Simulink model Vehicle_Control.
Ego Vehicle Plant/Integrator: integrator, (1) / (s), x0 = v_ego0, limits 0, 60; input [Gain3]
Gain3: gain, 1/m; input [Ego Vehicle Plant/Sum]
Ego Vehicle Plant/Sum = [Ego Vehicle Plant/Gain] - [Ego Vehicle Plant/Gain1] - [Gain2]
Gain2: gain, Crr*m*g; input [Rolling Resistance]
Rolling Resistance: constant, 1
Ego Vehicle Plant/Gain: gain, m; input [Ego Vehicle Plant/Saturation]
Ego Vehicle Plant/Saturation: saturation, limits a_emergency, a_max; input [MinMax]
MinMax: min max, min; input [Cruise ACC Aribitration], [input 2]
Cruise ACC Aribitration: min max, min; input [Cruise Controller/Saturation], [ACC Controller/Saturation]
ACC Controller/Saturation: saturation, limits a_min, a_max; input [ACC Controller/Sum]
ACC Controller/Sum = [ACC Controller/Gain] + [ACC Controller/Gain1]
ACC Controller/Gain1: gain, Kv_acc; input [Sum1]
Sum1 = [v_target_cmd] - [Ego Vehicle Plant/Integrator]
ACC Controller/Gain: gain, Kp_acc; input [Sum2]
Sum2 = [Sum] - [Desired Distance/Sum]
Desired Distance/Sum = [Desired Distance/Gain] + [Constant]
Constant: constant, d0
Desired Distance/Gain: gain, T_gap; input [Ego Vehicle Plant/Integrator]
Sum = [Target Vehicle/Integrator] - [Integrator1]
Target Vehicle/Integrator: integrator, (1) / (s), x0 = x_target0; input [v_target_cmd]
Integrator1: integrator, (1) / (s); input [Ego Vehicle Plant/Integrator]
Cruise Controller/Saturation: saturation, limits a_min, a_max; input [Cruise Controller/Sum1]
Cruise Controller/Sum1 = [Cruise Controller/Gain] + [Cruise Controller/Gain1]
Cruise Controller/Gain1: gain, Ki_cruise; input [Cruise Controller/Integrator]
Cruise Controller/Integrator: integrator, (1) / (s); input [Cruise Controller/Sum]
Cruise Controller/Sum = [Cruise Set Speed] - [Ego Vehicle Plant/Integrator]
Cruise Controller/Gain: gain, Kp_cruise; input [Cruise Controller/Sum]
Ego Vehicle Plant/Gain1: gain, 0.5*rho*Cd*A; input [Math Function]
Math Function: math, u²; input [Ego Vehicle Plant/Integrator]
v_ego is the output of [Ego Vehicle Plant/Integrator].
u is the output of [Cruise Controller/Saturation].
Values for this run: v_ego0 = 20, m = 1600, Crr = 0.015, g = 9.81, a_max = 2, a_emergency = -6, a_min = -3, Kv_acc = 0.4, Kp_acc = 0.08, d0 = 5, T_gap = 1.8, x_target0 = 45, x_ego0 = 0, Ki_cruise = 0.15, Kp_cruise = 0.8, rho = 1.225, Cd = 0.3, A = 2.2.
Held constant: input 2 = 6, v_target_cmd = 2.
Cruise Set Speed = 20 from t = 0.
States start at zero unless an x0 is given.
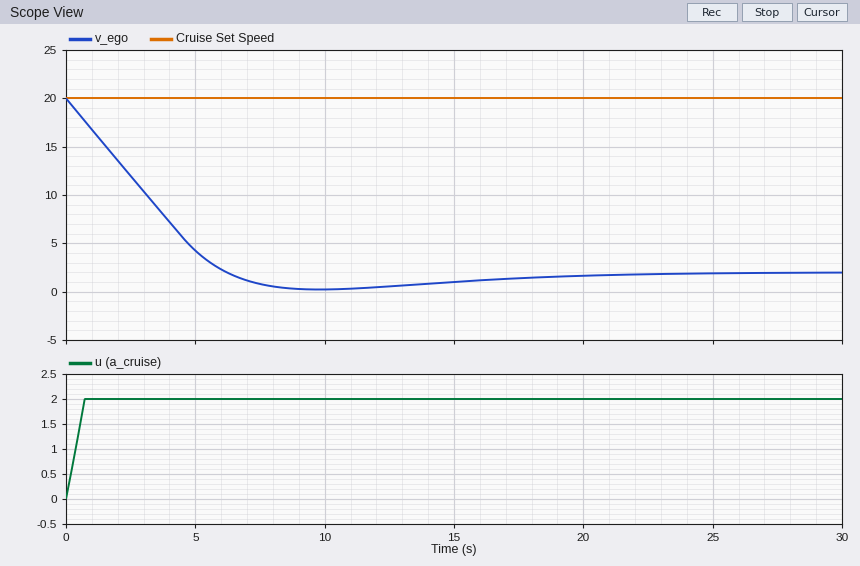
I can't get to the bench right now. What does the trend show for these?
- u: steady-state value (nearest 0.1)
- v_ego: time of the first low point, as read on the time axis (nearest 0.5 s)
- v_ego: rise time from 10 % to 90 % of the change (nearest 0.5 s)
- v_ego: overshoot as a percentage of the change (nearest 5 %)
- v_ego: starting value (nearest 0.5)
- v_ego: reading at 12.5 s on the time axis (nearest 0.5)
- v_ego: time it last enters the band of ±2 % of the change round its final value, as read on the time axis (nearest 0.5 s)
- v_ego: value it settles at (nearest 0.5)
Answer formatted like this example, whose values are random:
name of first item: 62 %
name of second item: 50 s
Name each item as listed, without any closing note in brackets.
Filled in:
u: steady-state value: 2.0
v_ego: time of the first low point, as read on the time axis: 10.0 s
v_ego: rise time from 10 % to 90 % of the change: 4.5 s
v_ego: overshoot as a percentage of the change: 10 %
v_ego: starting value: 20.0
v_ego: reading at 12.5 s on the time axis: 0.5
v_ego: time it last enters the band of ±2 % of the change round its final value, as read on the time axis: 20.0 s
v_ego: value it settles at: 2.0
